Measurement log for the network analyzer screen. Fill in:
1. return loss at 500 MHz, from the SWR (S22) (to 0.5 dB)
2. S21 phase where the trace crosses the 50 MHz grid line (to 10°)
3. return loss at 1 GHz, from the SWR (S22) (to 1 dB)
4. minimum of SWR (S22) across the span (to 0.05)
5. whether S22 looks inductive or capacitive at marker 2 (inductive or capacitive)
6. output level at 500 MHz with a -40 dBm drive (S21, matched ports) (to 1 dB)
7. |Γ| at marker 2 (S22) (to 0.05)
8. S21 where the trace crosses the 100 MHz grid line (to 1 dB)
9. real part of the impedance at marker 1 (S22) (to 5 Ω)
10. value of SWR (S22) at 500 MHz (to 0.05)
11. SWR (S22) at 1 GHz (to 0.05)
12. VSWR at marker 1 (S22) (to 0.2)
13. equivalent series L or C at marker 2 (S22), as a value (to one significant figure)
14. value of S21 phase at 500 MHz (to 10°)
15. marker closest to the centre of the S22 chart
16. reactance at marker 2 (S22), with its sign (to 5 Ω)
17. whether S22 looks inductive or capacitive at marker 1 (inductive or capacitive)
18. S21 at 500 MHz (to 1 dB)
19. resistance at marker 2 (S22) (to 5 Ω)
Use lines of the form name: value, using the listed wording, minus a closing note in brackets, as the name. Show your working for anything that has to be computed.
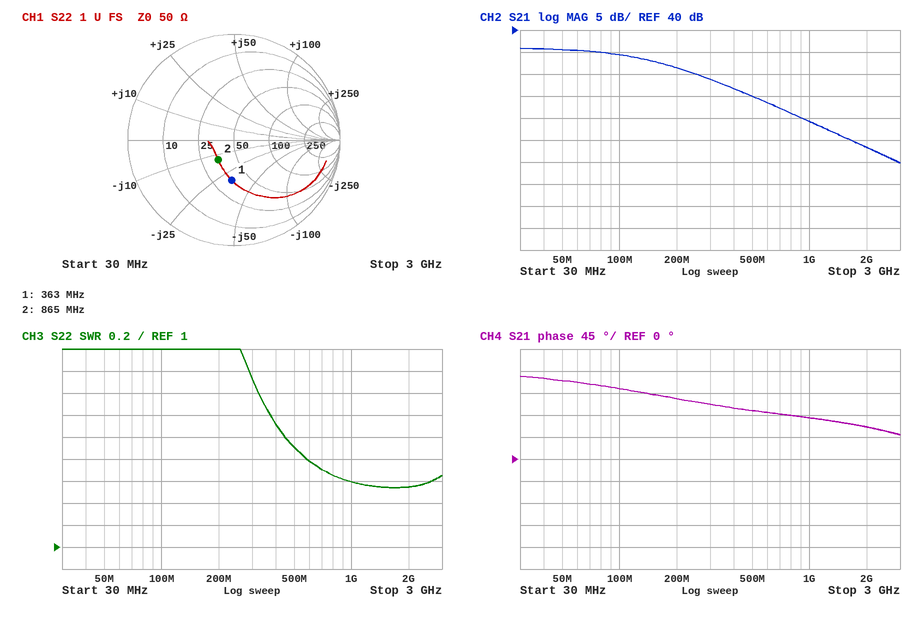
return loss at 500 MHz, from the SWR (S22): −20 log10((1.9 − 1)/(1.9 + 1)) ≈ 10.2 dB, so 10.0 dB to the nearest 0.5 dB
S21 phase where the trace crosses the 50 MHz grid line: 160°
return loss at 1 GHz, from the SWR (S22): −20 log10((1.6 − 1)/(1.6 + 1)) ≈ 13 dB
minimum of SWR (S22) across the span: 1.55
whether S22 looks inductive or capacitive at marker 2: capacitive
output level at 500 MHz with a -40 dBm drive (S21, matched ports): -40 dBm + (25 dB) = -15 dBm
|Γ| at marker 2 (S22): 0.25
S21 where the trace crosses the 100 MHz grid line: 34 dB
real part of the impedance at marker 1 (S22): 35 Ω
value of SWR (S22) at 500 MHz: 1.90
SWR (S22) at 1 GHz: 1.60
VSWR at marker 1 (S22): 2.2
equivalent series L or C at marker 2 (S22), as a value: C = 1/(2π × 865 MHz × 15 Ω) ≈ 12.3 pF, so 10 pF to one significant figure
value of S21 phase at 500 MHz: 100°
marker closest to the centre of the S22 chart: marker 2
reactance at marker 2 (S22), with its sign: -15 Ω
whether S22 looks inductive or capacitive at marker 1: capacitive
S21 at 500 MHz: 25 dB
resistance at marker 2 (S22): 35 Ω
